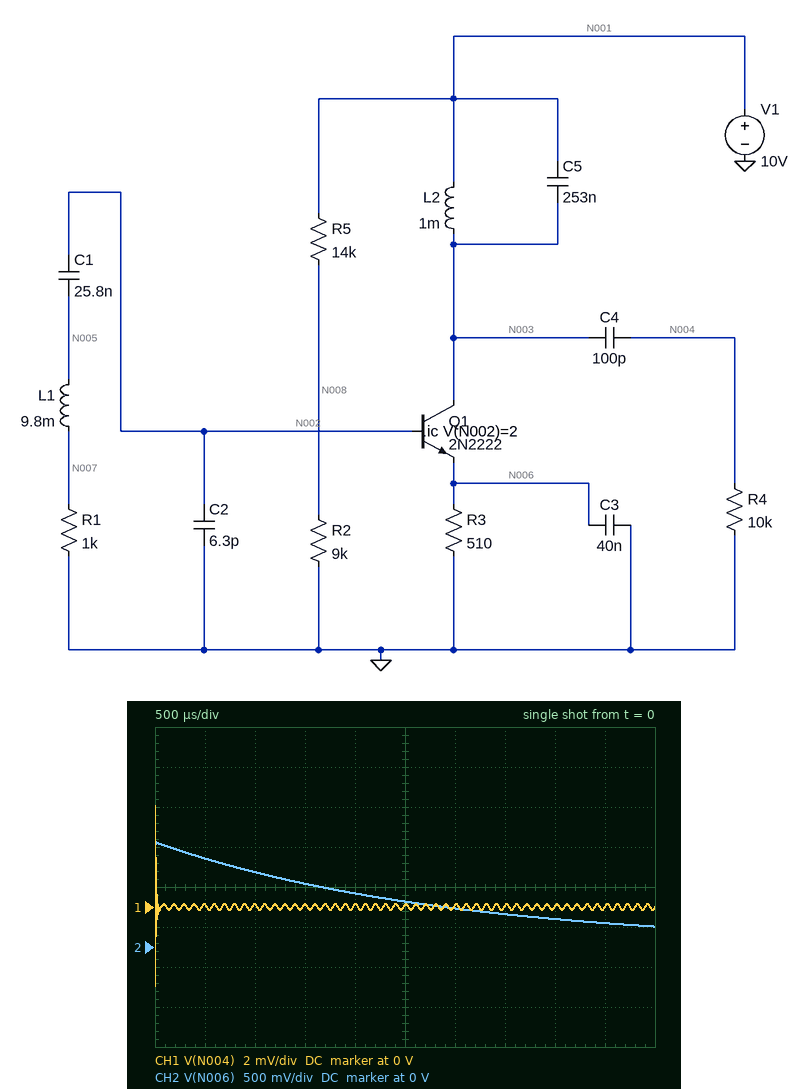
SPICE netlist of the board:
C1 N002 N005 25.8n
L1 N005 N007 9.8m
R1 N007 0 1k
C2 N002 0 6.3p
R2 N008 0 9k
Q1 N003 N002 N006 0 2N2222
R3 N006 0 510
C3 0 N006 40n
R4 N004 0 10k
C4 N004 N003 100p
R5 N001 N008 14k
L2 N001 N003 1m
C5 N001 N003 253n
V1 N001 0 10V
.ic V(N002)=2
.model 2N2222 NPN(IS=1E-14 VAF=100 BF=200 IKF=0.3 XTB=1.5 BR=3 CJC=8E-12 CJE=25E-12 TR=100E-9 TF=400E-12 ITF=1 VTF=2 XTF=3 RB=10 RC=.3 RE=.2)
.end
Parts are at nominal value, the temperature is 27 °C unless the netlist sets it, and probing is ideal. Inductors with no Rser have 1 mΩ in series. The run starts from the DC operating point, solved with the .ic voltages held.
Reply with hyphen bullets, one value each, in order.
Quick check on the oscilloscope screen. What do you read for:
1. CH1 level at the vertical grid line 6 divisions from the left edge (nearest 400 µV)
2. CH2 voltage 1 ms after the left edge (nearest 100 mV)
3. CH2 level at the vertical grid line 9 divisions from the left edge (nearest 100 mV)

- 0 V
- 900 mV
- 300 mV
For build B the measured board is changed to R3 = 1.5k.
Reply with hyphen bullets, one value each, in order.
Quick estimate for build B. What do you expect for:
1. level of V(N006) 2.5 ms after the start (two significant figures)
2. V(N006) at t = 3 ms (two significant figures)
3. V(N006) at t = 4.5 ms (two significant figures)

- 1.0 V
- 950 mV
- 800 mV
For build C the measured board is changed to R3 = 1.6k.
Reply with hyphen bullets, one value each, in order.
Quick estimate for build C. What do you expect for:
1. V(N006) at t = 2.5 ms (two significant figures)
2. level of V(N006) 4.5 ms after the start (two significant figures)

- 1.0 V
- 830 mV
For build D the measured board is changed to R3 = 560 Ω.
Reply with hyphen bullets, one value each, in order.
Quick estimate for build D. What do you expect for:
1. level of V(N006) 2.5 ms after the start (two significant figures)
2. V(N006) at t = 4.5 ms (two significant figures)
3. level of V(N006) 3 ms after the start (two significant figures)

- 610 mV
- 340 mV
- 530 mV
